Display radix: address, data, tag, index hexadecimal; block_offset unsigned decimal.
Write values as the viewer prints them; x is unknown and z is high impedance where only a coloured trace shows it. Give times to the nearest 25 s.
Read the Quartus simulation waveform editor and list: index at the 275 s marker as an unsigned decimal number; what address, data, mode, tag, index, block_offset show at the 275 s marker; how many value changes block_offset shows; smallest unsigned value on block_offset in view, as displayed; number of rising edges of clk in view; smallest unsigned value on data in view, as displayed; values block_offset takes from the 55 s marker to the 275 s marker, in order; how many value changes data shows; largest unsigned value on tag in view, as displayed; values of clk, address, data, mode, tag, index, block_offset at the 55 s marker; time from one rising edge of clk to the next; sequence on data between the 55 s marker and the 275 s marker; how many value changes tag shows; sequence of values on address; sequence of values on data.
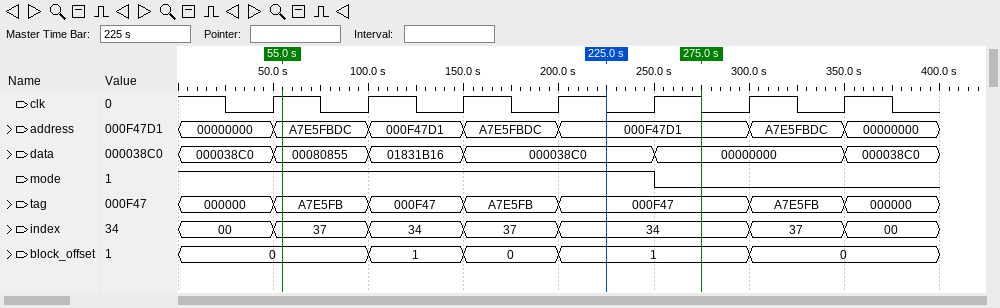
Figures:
52
address=000F47D1, data=00000000, mode=0, tag=000F47, index=34, block_offset=1
4
0
7
00000000
0, 1, 0, 1
5
A7E5FB
clk=1, address=A7E5FBDC, data=00080855, mode=1, tag=A7E5FB, index=37, block_offset=0
50 s
00080855, 01831B16, 000038C0, 00000000
6
00000000, A7E5FBDC, 000F47D1, A7E5FBDC, 000F47D1, A7E5FBDC, 00000000
000038C0, 00080855, 01831B16, 000038C0, 00000000, 000038C0
